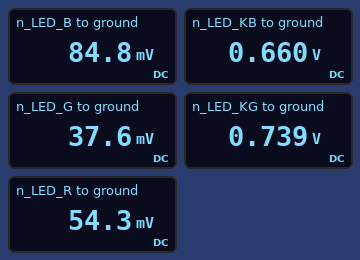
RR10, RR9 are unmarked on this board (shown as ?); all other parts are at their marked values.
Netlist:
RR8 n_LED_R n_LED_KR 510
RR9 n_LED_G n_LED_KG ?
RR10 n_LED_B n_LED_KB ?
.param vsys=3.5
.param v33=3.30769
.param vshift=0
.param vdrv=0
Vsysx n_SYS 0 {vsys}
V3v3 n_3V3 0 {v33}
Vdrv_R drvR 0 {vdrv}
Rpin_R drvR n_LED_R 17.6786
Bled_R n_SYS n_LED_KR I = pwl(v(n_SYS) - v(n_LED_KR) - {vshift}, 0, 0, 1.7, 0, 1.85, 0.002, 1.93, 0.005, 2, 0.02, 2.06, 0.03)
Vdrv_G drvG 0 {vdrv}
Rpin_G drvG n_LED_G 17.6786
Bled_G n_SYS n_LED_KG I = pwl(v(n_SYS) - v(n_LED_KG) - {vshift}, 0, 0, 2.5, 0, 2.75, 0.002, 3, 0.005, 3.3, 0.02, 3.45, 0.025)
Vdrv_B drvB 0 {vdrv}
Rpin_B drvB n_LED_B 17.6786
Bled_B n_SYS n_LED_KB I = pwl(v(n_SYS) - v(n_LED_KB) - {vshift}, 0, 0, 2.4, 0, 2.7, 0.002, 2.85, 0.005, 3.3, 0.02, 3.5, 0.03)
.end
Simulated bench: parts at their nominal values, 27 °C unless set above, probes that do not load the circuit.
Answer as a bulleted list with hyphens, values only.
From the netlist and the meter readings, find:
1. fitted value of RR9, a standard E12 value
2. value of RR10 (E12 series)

- 330 Ω
- 120 Ω
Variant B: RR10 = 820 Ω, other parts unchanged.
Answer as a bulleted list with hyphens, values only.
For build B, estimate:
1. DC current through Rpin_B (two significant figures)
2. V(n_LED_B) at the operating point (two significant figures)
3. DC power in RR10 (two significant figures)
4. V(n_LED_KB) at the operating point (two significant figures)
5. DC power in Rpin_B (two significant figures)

- 1.1 mA
- 20 mV
- 1.0 mW
- 930 mV
- 22 µW
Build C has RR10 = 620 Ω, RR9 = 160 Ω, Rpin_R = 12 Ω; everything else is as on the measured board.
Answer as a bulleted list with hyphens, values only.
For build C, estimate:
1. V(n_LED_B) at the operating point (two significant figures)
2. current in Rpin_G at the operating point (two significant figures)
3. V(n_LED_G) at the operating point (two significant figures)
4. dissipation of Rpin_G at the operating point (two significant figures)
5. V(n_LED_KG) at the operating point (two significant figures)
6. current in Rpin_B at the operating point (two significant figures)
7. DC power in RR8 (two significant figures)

- 25 mV
- 3.5 mA
- 62 mV
- 220 µW
- 620 mV
- 1.4 mA
- 4.9 mW
